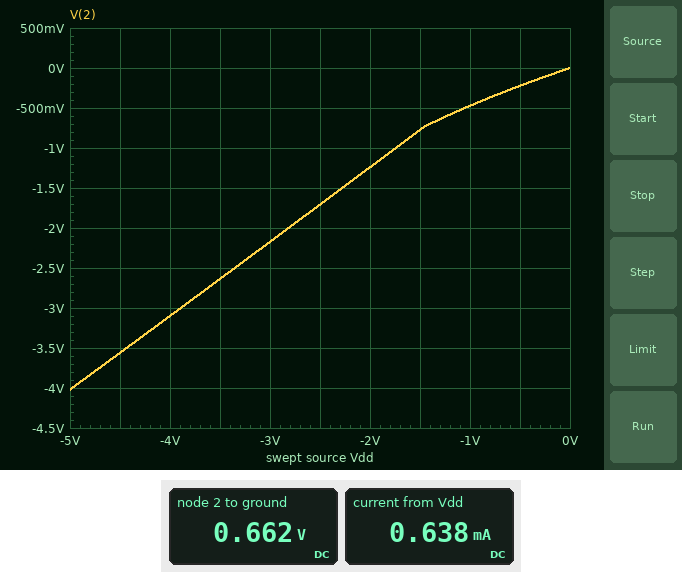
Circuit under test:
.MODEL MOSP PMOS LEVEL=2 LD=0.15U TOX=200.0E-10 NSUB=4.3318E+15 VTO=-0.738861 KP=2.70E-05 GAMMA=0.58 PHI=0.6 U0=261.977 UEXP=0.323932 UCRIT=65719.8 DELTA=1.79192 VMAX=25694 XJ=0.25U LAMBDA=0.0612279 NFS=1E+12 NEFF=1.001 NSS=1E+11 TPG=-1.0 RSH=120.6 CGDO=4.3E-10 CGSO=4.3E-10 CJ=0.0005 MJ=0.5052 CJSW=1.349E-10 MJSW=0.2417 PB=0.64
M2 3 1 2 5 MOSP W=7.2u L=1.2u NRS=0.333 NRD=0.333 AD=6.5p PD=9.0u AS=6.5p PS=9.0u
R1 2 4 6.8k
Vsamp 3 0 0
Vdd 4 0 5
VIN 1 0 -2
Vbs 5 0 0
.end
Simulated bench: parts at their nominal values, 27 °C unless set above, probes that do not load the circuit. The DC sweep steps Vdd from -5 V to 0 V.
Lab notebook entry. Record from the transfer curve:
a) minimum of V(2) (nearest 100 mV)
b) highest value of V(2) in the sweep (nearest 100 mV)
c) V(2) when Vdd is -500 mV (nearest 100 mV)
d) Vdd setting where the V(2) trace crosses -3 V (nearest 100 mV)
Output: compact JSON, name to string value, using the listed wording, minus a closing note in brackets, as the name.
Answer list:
{"minimum of V(2)": "-4.0 V", "highest value of V(2) in the sweep": "0 V", "V(2) when Vdd is -500 mV": "-200 mV", "Vdd setting where the V(2) trace crosses -3 V": "-3.9 V"}
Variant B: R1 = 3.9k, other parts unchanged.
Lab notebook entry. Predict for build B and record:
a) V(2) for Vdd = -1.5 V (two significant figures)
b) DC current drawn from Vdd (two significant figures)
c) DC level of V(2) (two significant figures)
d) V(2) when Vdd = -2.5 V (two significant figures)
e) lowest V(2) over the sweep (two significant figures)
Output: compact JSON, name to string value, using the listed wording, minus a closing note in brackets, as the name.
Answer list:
{"V(2) for Vdd = -1.5 V": "-1.1 V", "DC current drawn from Vdd": "1.1 mA", "DC level of V(2)": "700 mV", "V(2) when Vdd = -2.5 V": "-2.0 V", "lowest V(2) over the sweep": "-4.4 V"}
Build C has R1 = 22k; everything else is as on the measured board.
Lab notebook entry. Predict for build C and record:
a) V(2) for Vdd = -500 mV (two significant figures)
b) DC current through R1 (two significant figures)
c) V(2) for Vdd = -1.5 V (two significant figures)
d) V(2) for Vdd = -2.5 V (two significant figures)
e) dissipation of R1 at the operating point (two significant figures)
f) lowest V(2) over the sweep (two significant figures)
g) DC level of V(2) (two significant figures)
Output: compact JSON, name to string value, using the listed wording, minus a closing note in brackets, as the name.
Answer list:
{"V(2) for Vdd = -500 mV": "-96 mV", "DC current through R1": "200 µA", "V(2) for Vdd = -1.5 V": "-310 mV", "V(2) for Vdd = -2.5 V": "-560 mV", "dissipation of R1 at the operating point": "880 µW", "lowest V(2) over the sweep": "-2.3 V", "DC level of V(2)": "590 mV"}
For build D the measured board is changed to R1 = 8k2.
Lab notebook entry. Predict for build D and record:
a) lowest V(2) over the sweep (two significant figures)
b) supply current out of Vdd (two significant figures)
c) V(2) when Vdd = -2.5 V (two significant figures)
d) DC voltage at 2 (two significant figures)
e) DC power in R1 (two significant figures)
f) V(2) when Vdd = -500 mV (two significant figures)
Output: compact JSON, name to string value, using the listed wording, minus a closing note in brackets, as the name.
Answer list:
{"lowest V(2) over the sweep": "-3.8 V", "supply current out of Vdd": "530 µA", "V(2) when Vdd = -2.5 V": "-1.6 V", "DC voltage at 2": "650 mV", "DC power in R1": "2.3 mW", "V(2) when Vdd = -500 mV": "-200 mV"}
